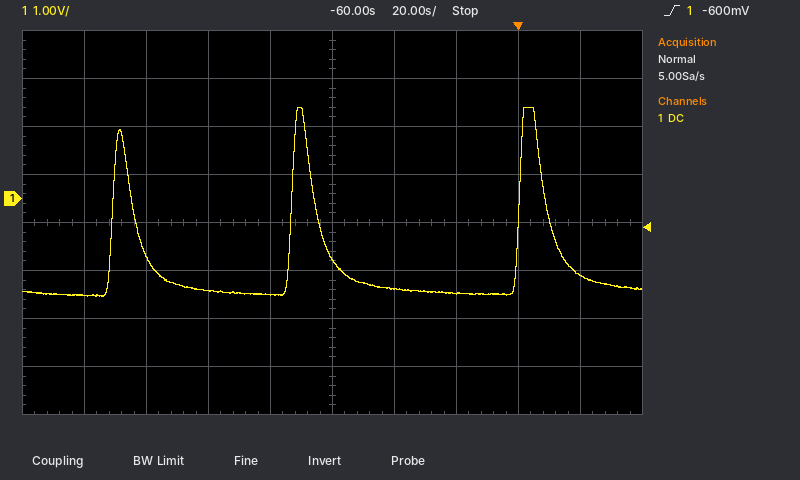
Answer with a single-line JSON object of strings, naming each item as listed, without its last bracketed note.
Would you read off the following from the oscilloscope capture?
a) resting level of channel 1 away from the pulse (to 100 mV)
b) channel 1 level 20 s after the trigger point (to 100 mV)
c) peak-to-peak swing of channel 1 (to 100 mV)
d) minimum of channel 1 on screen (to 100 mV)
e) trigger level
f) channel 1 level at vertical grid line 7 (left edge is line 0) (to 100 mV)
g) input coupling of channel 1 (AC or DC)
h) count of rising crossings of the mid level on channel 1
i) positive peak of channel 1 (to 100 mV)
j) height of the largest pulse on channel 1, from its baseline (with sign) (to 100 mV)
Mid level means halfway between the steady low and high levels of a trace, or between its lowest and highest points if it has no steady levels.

{"resting level of channel 1 away from the pulse": "-1.9 V", "channel 1 level 20 s after the trigger point": "-1.6 V", "peak-to-peak swing of channel 1": "3.9 V", "minimum of channel 1 on screen": "-2.0 V", "trigger level": "-600 mV", "channel 1 level at vertical grid line 7 (left edge is line 0)": "-2.0 V", "input coupling of channel 1": "DC", "count of rising crossings of the mid level on channel 1": "3", "positive peak of channel 1": "1.9 V", "height of the largest pulse on channel 1, from its baseline (with sign)": "+3.8 V"}
